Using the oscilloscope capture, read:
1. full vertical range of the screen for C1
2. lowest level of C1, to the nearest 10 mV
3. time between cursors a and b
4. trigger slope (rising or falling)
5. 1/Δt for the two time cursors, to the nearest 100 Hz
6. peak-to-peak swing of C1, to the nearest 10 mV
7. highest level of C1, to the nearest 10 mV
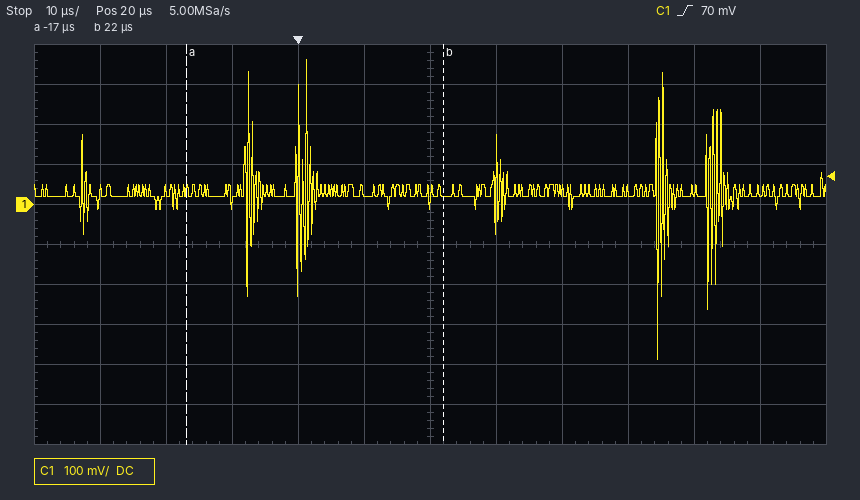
1 V
-390 mV
39 µs
rising
25.6 kHz
750 mV
360 mV
